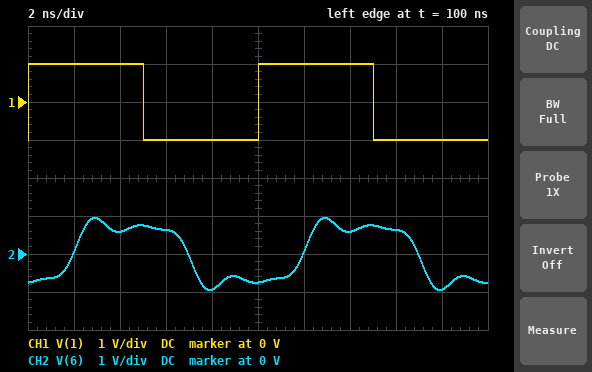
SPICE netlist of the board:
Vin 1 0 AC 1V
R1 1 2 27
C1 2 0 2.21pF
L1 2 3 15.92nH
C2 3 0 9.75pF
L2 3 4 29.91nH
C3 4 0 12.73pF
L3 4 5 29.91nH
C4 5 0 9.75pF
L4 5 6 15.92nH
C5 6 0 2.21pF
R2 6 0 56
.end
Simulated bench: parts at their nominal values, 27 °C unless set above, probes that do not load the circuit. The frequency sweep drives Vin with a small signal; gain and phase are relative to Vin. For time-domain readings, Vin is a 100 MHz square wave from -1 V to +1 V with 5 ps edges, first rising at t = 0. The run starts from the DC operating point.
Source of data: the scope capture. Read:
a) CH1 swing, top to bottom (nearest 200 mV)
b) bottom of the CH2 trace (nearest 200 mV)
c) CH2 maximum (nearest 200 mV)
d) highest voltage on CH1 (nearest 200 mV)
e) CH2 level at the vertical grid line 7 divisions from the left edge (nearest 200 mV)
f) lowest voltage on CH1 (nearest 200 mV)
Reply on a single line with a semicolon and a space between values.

2.0 V; -1.0 V; 1.0 V; 1.0 V; 600 mV; -1.0 V
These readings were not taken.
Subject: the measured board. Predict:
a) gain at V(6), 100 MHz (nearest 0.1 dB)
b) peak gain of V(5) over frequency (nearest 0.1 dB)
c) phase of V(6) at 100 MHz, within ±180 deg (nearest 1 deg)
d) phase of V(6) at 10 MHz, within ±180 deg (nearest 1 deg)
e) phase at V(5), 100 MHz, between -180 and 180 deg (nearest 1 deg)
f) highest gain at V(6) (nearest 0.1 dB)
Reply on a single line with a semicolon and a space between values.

-3.2 dB; -2.9 dB; -66 deg; -6 deg; -55 deg; -3.1 dB
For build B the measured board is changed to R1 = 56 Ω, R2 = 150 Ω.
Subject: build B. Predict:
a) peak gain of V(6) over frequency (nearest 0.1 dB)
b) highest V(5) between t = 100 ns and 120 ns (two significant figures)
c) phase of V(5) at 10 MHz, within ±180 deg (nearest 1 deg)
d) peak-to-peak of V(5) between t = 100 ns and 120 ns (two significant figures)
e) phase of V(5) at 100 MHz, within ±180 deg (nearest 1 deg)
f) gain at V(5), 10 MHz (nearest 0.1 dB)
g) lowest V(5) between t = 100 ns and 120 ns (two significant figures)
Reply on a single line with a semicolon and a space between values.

-2.5 dB; 870 mV; -7 deg; 1.7 V; -64 deg; -2.8 dB; -870 mV
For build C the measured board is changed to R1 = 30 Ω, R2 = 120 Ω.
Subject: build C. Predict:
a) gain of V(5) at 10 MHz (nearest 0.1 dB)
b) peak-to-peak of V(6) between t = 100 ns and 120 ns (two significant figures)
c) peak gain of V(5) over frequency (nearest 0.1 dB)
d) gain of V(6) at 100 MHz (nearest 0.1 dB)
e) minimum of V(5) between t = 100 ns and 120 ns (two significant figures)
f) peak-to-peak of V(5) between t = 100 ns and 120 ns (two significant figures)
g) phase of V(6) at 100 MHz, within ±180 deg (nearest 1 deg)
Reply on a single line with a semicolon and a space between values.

-1.9 dB; 2.6 V; -0.3 dB; -0.5 dB; -1.2 V; 2.4 V; -62 deg
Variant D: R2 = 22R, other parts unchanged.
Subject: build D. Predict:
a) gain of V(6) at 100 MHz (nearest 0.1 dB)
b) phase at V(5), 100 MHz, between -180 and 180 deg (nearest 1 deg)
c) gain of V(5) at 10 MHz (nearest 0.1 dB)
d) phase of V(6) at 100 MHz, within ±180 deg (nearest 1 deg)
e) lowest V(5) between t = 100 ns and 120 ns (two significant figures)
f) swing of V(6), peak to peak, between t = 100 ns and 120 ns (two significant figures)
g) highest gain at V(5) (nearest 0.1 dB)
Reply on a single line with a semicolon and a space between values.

-8.7 dB; -46 deg; -7.0 dB; -71 deg; -840 mV; 1.0 V; -0.2 dB
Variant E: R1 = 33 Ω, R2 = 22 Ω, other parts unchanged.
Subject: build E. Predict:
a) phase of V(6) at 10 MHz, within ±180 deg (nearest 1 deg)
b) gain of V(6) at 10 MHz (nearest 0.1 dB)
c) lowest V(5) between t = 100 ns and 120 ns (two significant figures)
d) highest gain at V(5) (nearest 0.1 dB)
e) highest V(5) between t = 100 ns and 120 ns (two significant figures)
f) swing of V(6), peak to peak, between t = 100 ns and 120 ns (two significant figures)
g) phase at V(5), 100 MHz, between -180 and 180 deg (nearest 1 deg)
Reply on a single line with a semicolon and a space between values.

-8 deg; -8.0 dB; -780 mV; -1.5 dB; 780 mV; 960 mV; -45 deg
